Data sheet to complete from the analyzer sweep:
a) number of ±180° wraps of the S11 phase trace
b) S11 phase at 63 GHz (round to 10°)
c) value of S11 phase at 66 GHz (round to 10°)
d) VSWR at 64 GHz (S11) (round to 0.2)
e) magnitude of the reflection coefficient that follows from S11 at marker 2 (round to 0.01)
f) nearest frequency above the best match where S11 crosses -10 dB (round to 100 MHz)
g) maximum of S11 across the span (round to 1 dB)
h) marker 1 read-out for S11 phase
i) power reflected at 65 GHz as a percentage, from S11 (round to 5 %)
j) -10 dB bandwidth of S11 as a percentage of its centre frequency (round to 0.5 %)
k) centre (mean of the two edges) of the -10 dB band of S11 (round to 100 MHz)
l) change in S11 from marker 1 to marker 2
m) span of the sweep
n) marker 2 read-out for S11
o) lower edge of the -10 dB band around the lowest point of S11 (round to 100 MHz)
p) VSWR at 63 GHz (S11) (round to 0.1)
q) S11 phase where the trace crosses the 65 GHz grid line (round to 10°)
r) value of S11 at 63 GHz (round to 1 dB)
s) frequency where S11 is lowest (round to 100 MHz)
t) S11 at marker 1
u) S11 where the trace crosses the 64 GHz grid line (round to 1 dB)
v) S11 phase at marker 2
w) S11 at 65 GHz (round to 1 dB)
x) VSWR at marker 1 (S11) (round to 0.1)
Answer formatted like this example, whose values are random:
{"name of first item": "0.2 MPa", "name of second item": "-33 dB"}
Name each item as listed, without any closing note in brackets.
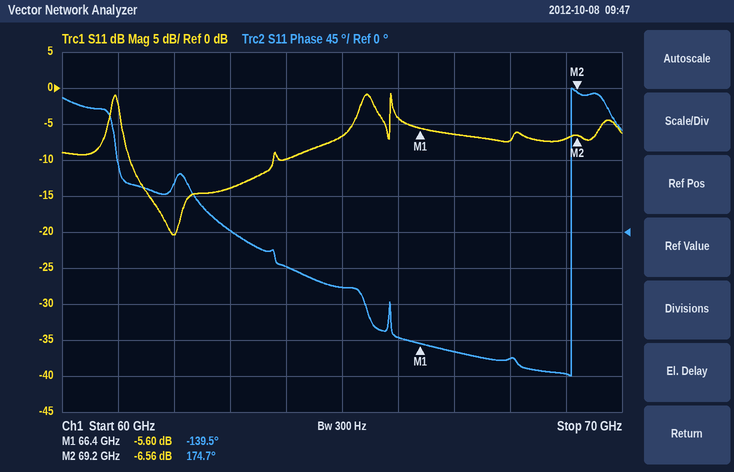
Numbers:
{"number of ±180° wraps of the S11 phase trace": "1", "S11 phase at 63 GHz": "0°", "value of S11 phase at 66 GHz": "-130°", "VSWR at 64 GHz (S11)": "2.0", "magnitude of the reflection coefficient that follows from S11 at marker 2": "0.47", "nearest frequency above the best match where S11 crosses -10 dB": "63.8 GHz", "maximum of S11 across the span": "-1 dB", "marker 1 read-out for S11 phase": "-139.5°", "power reflected at 65 GHz as a percentage, from S11": "20 %", "-10 dB bandwidth of S11 as a percentage of its centre frequency": "4.0 %", "centre (mean of the two edges) of the -10 dB band of S11": "62.5 GHz", "change in S11 from marker 1 to marker 2": "-0.96 dB", "span of the sweep": "10 GHz", "marker 2 read-out for S11": "-6.56 dB", "lower edge of the -10 dB band around the lowest point of S11": "61.2 GHz", "VSWR at 63 GHz (S11)": "1.5", "S11 phase where the trace crosses the 65 GHz grid line": "-70°", "value of S11 at 63 GHz": "-14 dB", "frequency where S11 is lowest": "62.0 GHz", "S11 at marker 1": "-5.60 dB", "S11 where the trace crosses the 64 GHz grid line": "-10 dB", "S11 phase at marker 2": "174.7°", "S11 at 65 GHz": "-7 dB", "VSWR at marker 1 (S11)": "3.2"}
